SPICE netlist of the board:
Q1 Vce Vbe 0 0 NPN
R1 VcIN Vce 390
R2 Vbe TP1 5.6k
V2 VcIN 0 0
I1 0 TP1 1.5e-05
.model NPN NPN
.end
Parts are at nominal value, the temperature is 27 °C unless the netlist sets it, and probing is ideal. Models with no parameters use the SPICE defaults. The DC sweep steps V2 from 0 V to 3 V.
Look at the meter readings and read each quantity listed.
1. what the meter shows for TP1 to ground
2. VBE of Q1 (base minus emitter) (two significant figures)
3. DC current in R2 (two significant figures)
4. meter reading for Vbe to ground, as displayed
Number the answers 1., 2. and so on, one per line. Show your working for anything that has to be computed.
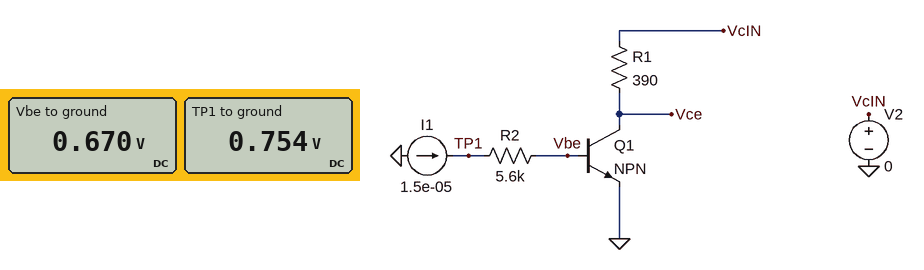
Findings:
1. 0.754 V
2. 670 mV = 670 mV
3. (754 mV - 670 mV) / 5.6 kΩ = 15 µA
4. 0.670 V
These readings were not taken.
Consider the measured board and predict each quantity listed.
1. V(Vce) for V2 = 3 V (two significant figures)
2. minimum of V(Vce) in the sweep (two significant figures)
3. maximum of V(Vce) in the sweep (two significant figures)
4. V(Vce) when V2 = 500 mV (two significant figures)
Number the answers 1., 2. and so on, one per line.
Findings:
1. 2.4 V
2. 4.6 mV
3. 2.4 V
4. 130 mV
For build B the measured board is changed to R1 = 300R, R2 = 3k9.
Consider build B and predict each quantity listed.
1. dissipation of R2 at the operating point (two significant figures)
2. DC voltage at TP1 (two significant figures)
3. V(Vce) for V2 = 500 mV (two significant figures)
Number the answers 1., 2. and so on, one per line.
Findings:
1. 880 nW
2. 730 mV
3. 150 mV
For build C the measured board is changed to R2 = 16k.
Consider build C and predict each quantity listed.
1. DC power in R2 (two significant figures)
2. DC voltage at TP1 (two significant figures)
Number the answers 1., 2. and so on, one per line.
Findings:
1. 3.6 µW
2. 910 mV
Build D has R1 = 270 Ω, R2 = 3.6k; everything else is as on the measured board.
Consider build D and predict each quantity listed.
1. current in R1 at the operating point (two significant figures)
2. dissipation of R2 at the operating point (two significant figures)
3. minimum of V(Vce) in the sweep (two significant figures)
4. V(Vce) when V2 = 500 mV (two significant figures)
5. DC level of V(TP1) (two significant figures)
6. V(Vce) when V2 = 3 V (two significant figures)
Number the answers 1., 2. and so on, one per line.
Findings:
1. 13 µA
2. 810 nW
3. 3.4 mV
4. 160 mV
5. 720 mV
6. 2.6 V
